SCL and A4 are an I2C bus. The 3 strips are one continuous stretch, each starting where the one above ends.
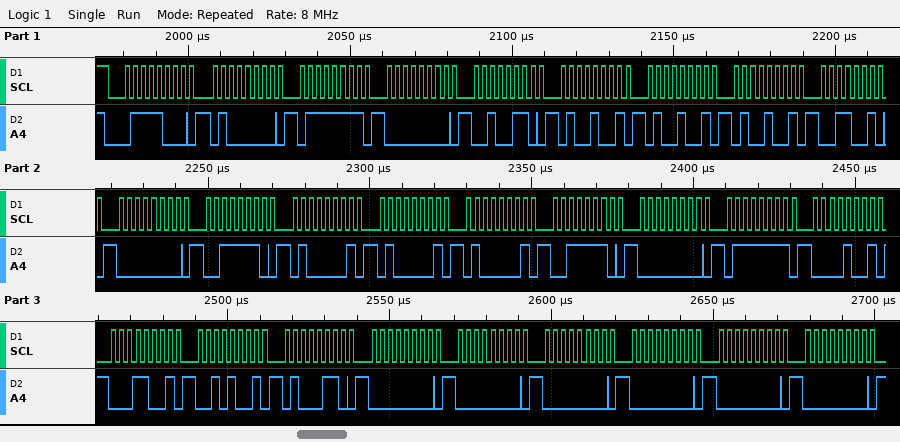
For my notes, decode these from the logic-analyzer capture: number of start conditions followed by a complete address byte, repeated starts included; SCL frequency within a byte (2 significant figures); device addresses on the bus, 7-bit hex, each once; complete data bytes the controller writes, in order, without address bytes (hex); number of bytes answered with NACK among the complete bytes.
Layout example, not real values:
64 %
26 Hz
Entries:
1
400 kHz
0x3C
40 7F 00 26 49 49 49 32 00 3E 41 41 41 3E 00 7F 09 19 29 46 00 00 00 00 00 00
0
